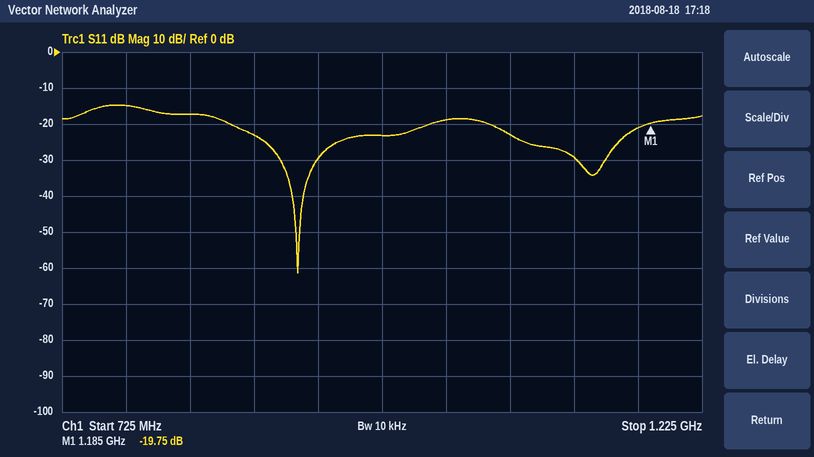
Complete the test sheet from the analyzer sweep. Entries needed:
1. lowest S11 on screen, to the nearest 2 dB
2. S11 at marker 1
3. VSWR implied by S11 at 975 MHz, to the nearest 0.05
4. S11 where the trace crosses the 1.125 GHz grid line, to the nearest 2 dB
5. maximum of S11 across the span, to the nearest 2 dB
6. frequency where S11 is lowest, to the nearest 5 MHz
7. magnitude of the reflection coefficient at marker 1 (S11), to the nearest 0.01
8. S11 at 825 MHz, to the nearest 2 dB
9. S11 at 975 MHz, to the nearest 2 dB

-62 dB
-19.75 dB
1.15
-30 dB
-14 dB
910 MHz
0.10
-18 dB
-24 dB
